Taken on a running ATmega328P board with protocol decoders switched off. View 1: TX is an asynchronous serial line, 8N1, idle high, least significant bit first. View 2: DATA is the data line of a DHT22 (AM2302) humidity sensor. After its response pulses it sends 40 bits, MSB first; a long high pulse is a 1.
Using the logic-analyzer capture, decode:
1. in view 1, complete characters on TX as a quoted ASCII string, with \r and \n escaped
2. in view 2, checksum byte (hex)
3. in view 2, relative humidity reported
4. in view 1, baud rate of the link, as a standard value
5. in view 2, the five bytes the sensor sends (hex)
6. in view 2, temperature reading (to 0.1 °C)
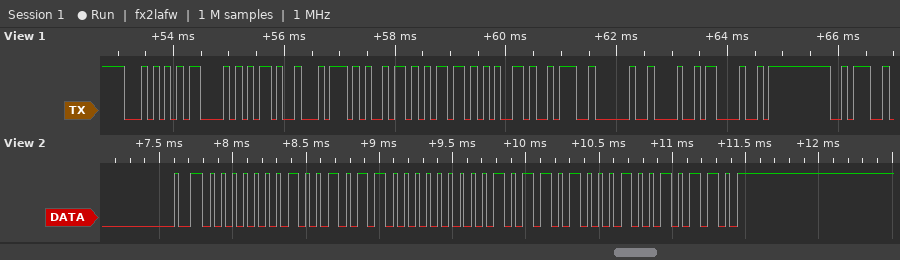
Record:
"TC-time: HH:"
0x96
30.0 %
9600 baud
01 2C 01 68 96
36.0 °C
